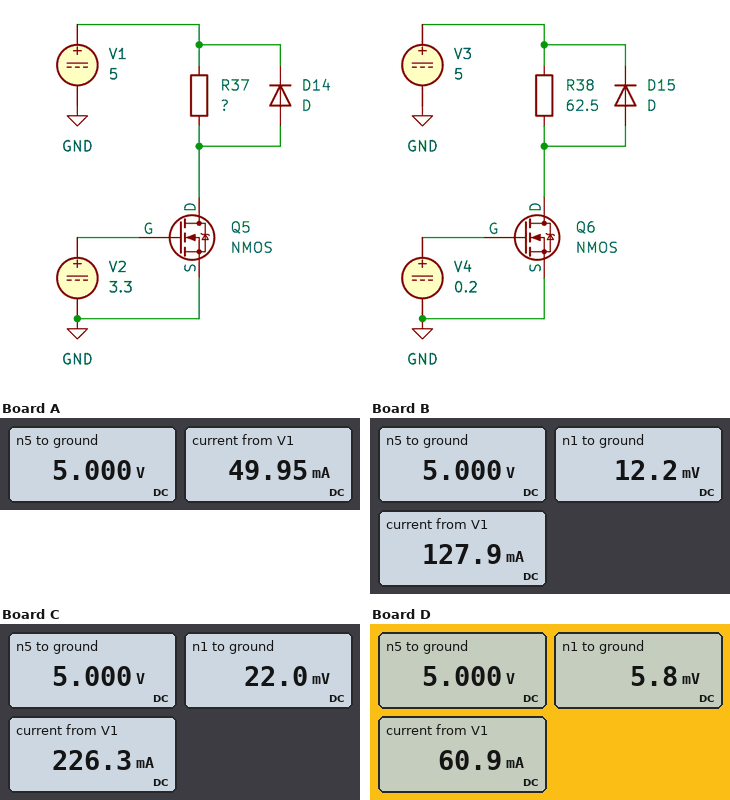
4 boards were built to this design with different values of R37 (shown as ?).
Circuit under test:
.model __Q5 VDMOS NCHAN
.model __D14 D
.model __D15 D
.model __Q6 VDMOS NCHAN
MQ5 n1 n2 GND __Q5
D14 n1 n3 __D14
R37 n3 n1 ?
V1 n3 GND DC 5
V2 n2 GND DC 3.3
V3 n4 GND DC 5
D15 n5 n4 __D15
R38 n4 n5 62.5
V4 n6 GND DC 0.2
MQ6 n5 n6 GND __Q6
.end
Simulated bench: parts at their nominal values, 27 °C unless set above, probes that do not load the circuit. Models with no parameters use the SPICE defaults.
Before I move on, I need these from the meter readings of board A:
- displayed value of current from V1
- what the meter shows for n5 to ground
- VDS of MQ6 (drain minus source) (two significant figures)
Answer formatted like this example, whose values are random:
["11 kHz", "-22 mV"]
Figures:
["49.95 mA", "5.000 V", "5.0 V"]
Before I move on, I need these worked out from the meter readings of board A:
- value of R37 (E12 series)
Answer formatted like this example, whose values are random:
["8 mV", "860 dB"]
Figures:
["100 Ω"]
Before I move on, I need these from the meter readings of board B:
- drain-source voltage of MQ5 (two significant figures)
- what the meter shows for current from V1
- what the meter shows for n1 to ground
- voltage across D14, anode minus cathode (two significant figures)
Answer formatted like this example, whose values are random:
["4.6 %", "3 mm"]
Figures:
["12 mV", "127.9 mA", "12.2 mV", "-5.0 V"]
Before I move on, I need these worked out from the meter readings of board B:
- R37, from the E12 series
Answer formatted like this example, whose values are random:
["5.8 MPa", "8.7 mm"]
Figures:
["39 Ω"]
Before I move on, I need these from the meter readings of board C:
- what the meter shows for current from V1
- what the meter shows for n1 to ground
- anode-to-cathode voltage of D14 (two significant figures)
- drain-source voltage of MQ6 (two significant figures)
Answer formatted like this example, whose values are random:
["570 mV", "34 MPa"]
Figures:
["226.3 mA", "22.0 mV", "-5.0 V", "5.0 V"]
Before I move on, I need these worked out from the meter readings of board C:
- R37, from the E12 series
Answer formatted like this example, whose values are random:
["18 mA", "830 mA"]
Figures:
["22 Ω"]
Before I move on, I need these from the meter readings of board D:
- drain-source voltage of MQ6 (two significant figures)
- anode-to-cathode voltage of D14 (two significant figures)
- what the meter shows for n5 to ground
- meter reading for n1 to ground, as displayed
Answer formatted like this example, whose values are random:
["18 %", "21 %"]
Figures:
["5.0 V", "-5.0 V", "5.000 V", "5.8 mV"]
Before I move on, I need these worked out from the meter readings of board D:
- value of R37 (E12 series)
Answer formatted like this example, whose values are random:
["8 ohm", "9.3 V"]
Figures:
["82 Ω"]
